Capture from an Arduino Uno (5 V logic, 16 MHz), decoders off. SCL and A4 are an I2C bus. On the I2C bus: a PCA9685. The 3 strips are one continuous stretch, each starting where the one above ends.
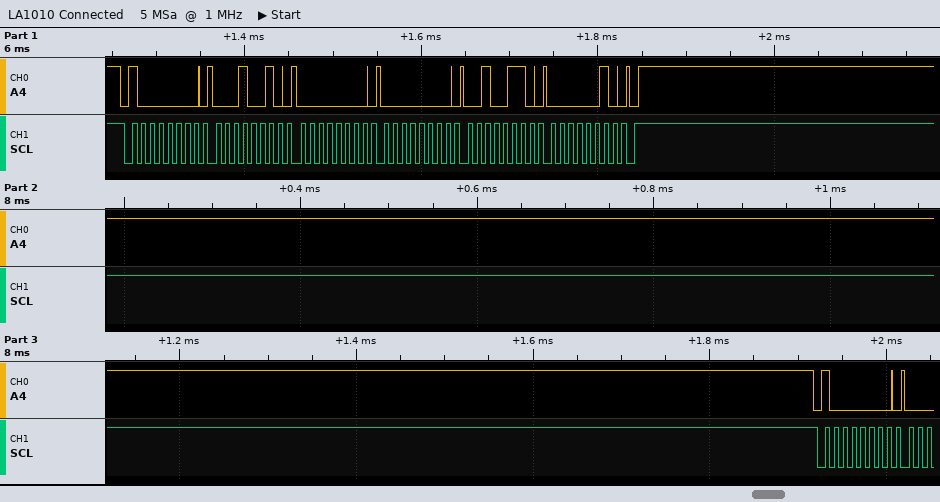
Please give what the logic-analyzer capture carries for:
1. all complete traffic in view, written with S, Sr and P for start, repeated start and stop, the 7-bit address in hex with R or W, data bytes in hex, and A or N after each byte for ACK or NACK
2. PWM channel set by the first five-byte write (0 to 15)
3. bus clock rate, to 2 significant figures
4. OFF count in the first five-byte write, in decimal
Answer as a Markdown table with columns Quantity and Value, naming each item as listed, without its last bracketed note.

| Quantity | Value |
|---|---|
| all complete traffic in view, written with S, Sr and P for start, repeated start and stop, the 7-bit address in hex with R or W, data bytes in hex, and A or N after each byte for ACK or NACK | S 40W A 12 A 00 A 00 A 26 A 02 A P S 40W A |
| PWM channel set by the first five-byte write | 3 |
| bus clock rate, to 2 significant figures | 100 kHz |
| OFF count in the first five-byte write, in decimal | 550 |
